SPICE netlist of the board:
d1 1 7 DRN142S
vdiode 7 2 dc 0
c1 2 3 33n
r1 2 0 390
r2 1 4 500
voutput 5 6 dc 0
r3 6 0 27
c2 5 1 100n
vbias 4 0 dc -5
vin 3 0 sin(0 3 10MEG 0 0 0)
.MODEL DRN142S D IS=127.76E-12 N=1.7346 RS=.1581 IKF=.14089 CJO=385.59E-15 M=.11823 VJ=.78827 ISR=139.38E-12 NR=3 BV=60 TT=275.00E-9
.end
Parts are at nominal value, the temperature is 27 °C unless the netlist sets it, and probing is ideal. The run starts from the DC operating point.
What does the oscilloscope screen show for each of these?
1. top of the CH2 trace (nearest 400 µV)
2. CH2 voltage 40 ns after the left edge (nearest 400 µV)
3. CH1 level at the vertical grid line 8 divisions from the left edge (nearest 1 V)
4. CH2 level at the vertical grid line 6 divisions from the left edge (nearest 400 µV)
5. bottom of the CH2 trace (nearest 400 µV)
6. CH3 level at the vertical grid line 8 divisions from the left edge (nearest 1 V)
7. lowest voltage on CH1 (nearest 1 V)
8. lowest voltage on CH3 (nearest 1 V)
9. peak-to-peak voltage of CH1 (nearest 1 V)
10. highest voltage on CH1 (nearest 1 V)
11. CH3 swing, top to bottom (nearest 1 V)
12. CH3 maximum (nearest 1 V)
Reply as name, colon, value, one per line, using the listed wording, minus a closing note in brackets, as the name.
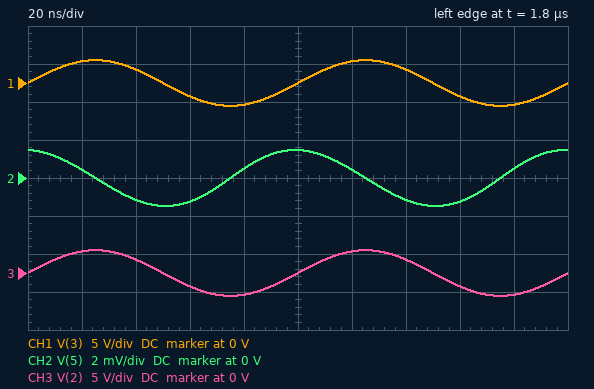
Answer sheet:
top of the CH2 trace: 1.6 mV
CH2 voltage 40 ns after the left edge: -1.2 mV
CH1 level at the vertical grid line 8 divisions from the left edge: -2 V
CH2 level at the vertical grid line 6 divisions from the left edge: 400 µV
bottom of the CH2 trace: -1.6 mV
CH3 level at the vertical grid line 8 divisions from the left edge: -2 V
lowest voltage on CH1: -3 V
lowest voltage on CH3: -3 V
peak-to-peak voltage of CH1: 6 V
highest voltage on CH1: 3 V
CH3 swing, top to bottom: 6 V
CH3 maximum: 3 V
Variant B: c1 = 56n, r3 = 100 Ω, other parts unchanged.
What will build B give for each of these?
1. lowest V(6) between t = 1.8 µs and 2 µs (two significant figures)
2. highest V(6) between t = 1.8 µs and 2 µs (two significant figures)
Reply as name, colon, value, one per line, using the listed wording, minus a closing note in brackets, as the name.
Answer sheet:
lowest V(6) between t = 1.8 µs and 2 µs: -4.8 mV
highest V(6) between t = 1.8 µs and 2 µs: 4.8 mV
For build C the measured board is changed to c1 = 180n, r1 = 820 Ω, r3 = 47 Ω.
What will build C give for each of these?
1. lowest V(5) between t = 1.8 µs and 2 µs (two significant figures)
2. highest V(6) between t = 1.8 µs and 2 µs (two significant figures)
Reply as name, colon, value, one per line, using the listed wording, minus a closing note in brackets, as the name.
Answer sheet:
lowest V(5) between t = 1.8 µs and 2 µs: -2.5 mV
highest V(6) between t = 1.8 µs and 2 µs: 2.5 mV
